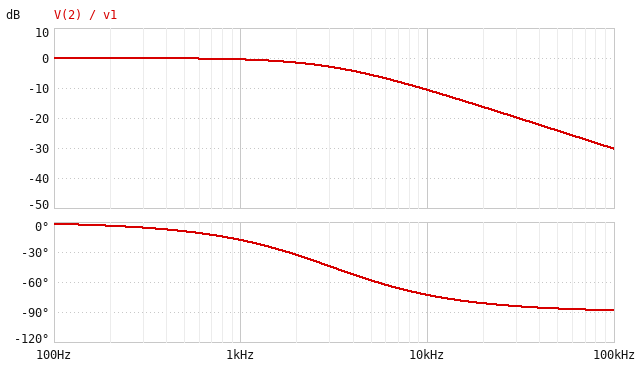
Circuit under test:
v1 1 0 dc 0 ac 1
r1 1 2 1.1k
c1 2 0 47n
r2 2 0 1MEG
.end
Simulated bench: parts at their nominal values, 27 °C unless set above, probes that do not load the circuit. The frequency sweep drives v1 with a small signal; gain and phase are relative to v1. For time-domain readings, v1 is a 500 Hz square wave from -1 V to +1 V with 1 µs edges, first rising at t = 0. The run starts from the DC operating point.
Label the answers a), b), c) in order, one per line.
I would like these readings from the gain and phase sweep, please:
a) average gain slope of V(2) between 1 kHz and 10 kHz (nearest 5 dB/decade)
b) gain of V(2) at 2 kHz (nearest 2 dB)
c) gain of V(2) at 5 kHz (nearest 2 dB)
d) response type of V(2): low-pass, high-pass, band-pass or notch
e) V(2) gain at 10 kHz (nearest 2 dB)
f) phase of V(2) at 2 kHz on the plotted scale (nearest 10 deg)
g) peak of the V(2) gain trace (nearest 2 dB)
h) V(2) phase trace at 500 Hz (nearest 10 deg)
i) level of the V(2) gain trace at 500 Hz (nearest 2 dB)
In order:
a) -10 dB/decade
b) -2 dB
c) -6 dB
d) low-pass
e) -10 dB
f) -30 deg
g) 0 dB
h) -10 deg
i) 0 dB
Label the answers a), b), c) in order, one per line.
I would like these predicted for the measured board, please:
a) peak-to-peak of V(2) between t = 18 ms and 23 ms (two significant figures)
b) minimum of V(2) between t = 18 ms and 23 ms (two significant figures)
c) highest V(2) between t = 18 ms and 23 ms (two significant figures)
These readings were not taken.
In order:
a) 2.0 V
b) -1.0 V
c) 1.0 V
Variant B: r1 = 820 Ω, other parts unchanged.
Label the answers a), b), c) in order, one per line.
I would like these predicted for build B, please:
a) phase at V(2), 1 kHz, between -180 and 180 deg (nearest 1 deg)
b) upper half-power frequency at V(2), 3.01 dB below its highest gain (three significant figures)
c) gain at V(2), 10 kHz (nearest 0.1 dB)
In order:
a) -14 deg
b) 4.13 kHz
c) -8.4 dB
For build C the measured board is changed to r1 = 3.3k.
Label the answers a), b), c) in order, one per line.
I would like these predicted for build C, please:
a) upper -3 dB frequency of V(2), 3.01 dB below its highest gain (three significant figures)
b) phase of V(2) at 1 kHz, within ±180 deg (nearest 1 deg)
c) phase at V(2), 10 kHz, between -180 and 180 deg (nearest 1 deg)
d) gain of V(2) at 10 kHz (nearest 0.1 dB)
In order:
a) 1.03 kHz
b) -44 deg
c) -84 deg
d) -19.8 dB
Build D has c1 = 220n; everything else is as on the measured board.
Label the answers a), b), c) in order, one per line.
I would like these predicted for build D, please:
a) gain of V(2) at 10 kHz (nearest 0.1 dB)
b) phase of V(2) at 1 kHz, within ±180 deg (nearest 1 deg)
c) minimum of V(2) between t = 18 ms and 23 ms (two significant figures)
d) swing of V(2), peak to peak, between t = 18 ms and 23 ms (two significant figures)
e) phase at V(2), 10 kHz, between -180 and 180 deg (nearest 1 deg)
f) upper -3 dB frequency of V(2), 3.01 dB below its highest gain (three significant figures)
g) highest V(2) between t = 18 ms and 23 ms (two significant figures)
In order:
a) -23.7 dB
b) -57 deg
c) -970 mV
d) 1.9 V
e) -86 deg
f) 658 Hz
g) 970 mV
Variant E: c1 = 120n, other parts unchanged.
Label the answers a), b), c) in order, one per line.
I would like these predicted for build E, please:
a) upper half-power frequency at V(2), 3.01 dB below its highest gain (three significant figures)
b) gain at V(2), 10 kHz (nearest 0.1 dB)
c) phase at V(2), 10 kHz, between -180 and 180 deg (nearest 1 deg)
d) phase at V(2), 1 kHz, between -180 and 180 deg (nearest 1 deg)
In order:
a) 1.21 kHz
b) -18.4 dB
c) -83 deg
d) -40 deg
